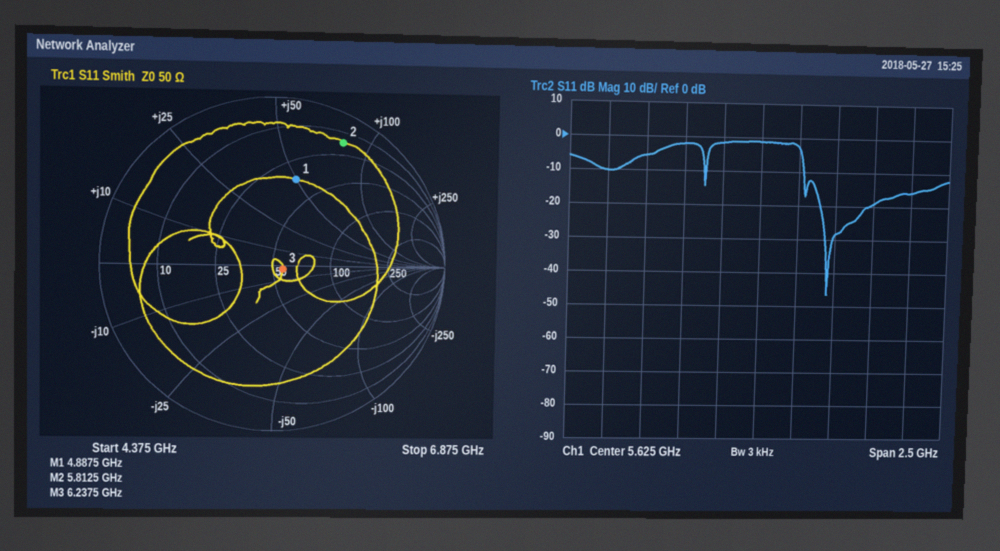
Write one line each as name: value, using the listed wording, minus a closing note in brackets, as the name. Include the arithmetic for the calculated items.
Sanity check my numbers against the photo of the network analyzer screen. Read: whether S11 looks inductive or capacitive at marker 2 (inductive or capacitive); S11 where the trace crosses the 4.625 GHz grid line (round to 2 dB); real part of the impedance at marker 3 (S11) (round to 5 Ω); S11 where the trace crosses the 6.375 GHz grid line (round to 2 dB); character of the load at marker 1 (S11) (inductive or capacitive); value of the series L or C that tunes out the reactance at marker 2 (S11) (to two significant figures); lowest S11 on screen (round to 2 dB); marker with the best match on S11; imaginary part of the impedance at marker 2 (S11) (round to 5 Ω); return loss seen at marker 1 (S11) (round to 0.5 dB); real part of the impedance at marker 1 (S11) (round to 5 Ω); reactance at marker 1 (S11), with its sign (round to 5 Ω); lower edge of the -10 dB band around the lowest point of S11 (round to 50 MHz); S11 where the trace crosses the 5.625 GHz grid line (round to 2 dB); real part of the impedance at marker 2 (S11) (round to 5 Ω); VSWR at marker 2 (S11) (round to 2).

whether S11 looks inductive or capacitive at marker 2: inductive
S11 where the trace crosses the 4.625 GHz grid line: -10 dB
real part of the impedance at marker 3 (S11): 55 Ω
S11 where the trace crosses the 6.375 GHz grid line: -20 dB
character of the load at marker 1 (S11): inductive
value of the series L or C that tunes out the reactance at marker 2 (S11): C = 1/(2π × 5.8125 GHz × 80 Ω) ≈ 342 fF, so 340 fF to two significant figures
lowest S11 on screen: -46 dB
marker with the best match on S11: marker 3
imaginary part of the impedance at marker 2 (S11): +80 Ω
return loss seen at marker 1 (S11): 5.5 dB
real part of the impedance at marker 1 (S11): 35 Ω
reactance at marker 1 (S11), with its sign: +50 Ω
lower edge of the -10 dB band around the lowest point of S11: 5.90 GHz
S11 where the trace crosses the 5.625 GHz grid line: -2 dB
real part of the impedance at marker 2 (S11): 15 Ω
VSWR at marker 2 (S11): 12
